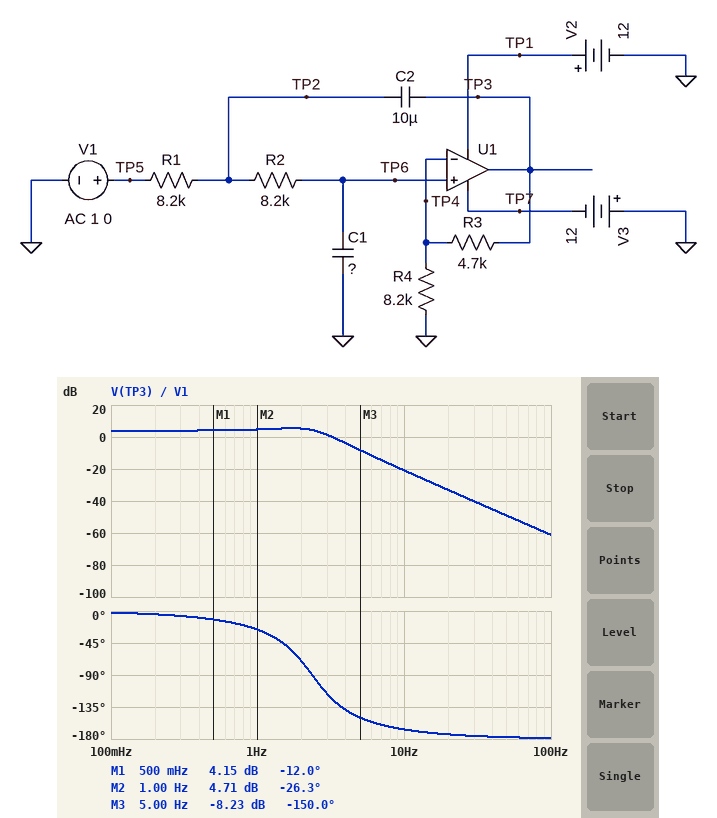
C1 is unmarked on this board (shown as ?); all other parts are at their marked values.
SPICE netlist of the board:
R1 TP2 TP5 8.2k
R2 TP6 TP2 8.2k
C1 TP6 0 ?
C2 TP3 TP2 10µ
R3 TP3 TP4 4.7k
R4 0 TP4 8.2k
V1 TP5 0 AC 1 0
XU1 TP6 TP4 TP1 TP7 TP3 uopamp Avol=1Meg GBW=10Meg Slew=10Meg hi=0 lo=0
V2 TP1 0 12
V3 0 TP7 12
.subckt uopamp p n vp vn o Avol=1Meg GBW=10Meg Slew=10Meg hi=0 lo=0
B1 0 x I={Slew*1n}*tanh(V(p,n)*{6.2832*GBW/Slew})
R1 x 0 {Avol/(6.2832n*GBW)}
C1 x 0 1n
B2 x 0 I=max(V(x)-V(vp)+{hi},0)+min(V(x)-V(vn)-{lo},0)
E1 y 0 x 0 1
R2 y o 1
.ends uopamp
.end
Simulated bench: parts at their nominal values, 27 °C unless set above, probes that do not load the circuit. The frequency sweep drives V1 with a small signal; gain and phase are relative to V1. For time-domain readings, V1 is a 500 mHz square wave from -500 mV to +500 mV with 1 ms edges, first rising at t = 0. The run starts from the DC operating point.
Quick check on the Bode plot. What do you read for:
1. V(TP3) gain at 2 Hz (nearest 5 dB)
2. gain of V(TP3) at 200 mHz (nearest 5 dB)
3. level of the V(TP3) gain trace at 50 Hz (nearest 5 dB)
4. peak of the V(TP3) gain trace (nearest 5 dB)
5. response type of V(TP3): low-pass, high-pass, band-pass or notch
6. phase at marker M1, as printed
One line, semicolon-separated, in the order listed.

5 dB; 5 dB; -50 dB; 5 dB; low-pass; -12.0 deg
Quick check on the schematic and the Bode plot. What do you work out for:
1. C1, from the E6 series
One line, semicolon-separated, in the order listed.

6.8 µF
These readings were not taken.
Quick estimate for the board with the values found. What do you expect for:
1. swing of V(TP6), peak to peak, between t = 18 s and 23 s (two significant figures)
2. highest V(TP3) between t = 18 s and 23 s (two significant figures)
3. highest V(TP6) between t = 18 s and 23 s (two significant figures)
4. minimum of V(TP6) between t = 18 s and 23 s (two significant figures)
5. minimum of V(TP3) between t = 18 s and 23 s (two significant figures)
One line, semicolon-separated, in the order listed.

1.4 V; 1.1 V; 680 mV; -680 mV; -1.1 V
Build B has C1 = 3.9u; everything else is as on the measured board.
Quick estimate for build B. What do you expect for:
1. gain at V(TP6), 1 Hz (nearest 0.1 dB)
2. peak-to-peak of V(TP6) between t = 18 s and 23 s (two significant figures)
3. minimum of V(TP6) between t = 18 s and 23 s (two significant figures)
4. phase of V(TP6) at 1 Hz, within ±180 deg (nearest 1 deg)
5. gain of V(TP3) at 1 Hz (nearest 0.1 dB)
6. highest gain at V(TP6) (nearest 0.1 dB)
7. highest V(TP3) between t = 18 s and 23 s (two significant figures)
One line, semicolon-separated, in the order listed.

0.9 dB; 2.1 V; -1.1 V; -7 deg; 4.8 dB; 9.7 dB; 1.7 V
